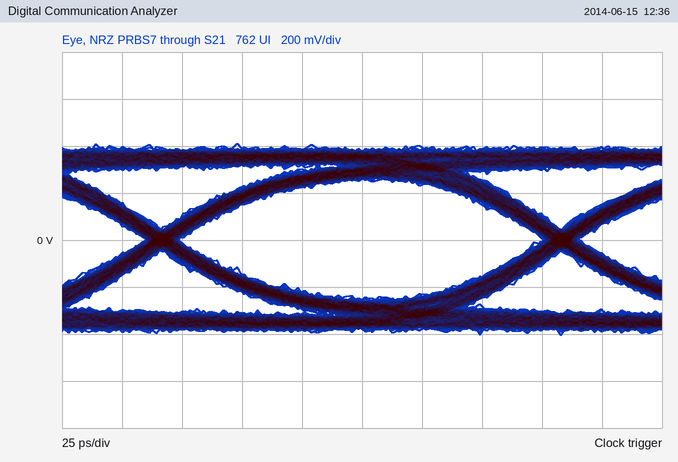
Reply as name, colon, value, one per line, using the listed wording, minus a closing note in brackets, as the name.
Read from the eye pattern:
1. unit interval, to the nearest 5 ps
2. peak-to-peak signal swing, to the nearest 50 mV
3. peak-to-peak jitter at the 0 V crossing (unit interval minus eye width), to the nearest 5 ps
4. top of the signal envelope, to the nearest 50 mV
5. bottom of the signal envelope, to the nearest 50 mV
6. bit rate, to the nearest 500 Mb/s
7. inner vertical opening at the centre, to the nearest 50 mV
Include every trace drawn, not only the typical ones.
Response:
unit interval, to the nearest 5 ps: 165 ps
peak-to-peak signal swing, to the nearest 50 mV: 800 mV
peak-to-peak jitter at the 0 V crossing (unit interval minus eye width), to the nearest 5 ps: 15 ps
top of the signal envelope, to the nearest 50 mV: 400 mV
bottom of the signal envelope, to the nearest 50 mV: -400 mV
bit rate, to the nearest 500 Mb/s: 6.0 Gb/s
inner vertical opening at the centre, to the nearest 50 mV: 500 mV
